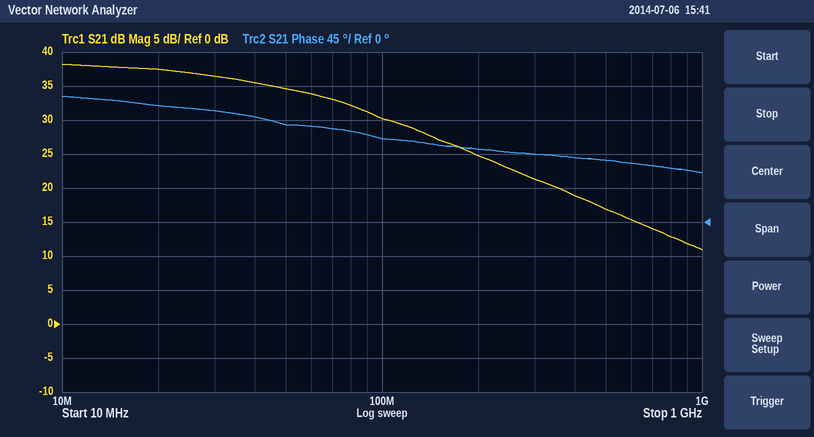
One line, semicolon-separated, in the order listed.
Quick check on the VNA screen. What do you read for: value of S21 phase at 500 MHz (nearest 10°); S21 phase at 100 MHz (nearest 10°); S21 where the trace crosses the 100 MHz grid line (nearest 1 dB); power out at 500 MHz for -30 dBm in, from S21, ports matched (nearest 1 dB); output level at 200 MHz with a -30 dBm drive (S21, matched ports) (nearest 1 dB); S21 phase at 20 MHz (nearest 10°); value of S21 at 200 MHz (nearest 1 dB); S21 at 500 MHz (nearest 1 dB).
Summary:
80°; 110°; 30 dB; -13 dBm; -5 dBm; 150°; 25 dB; 17 dB
